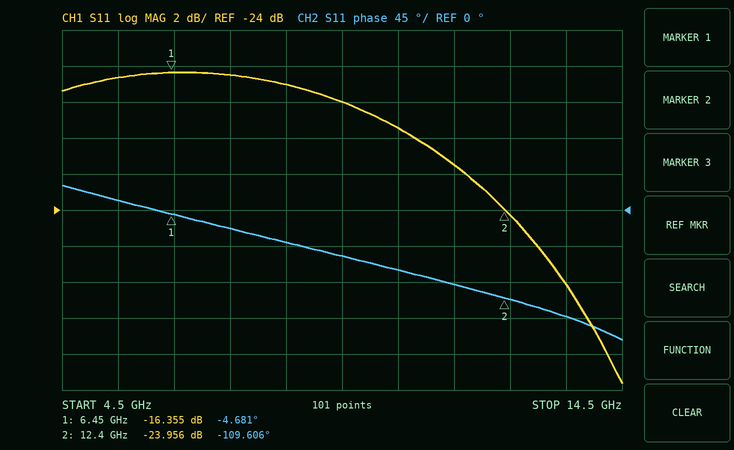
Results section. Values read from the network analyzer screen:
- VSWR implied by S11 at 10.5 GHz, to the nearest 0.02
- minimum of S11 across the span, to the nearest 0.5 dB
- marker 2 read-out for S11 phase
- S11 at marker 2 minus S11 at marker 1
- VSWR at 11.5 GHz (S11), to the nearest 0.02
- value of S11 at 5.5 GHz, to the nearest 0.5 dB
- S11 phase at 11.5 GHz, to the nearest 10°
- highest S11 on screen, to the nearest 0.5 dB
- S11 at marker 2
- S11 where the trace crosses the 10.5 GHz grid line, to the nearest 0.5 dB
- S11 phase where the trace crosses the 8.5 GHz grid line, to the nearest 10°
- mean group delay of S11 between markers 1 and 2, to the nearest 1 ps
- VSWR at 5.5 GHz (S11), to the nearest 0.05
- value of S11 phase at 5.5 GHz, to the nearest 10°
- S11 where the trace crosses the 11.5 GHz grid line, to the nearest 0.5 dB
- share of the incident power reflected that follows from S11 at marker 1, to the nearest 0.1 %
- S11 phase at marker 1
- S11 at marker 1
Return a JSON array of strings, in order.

["1.24", "-33.5 dB", "-109.606°", "-7.601 dB", "1.18", "-16.5 dB", "-90°", "-16.5 dB", "-23.956 dB", "-19.5 dB", "-40°", "49 ps", "1.35", "10°", "-21.5 dB", "2.3 %", "-4.681°", "-16.355 dB"]
